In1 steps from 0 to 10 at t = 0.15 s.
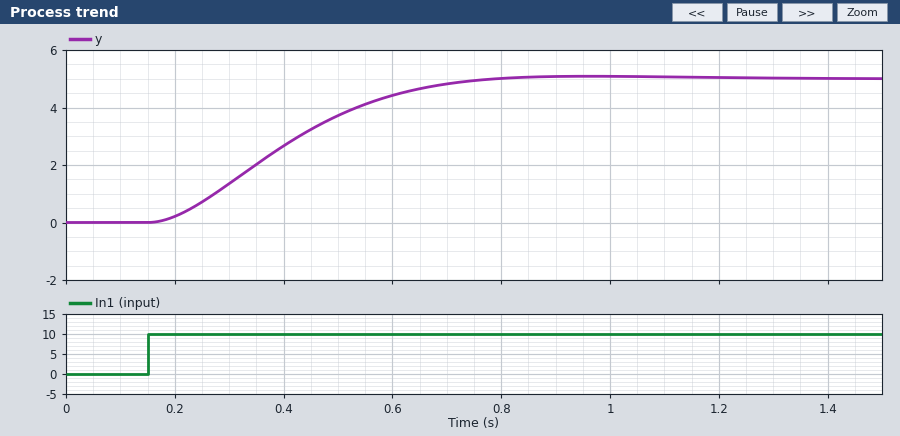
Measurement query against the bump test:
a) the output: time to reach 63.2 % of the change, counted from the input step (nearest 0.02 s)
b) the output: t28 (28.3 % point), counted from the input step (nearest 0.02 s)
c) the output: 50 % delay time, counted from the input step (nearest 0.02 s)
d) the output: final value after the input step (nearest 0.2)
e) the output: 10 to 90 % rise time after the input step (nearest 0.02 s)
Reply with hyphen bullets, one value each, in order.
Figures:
- 0.30 s
- 0.16 s
- 0.24 s
- 5.0
- 0.38 s
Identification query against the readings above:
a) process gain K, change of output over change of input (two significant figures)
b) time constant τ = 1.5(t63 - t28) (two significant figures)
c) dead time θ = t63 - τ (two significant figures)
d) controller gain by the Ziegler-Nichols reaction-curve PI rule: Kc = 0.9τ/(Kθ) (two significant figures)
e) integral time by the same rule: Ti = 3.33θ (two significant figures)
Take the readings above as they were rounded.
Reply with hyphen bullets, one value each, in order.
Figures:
- 0.50
- 0.21 s
- 0.090 s
- 4.2
- 0.30 s
